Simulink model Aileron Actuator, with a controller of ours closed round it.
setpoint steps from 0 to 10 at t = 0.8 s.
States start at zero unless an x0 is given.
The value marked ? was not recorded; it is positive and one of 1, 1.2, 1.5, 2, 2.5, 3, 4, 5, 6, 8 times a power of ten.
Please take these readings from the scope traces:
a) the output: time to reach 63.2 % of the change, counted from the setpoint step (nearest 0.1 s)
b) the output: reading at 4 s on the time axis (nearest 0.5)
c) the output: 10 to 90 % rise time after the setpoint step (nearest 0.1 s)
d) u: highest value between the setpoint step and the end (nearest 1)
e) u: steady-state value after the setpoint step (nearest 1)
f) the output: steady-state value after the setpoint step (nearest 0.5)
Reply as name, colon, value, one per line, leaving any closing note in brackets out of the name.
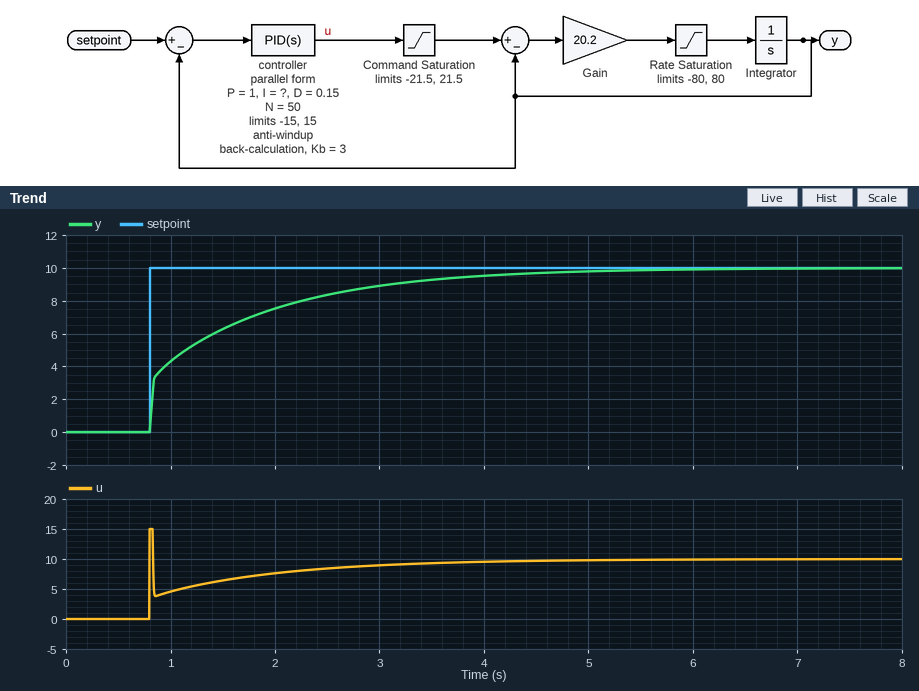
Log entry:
the output: time to reach 63.2 % of the change, counted from the setpoint step: 0.7 s
the output: reading at 4 s on the time axis: 9.5
the output: 10 to 90 % rise time after the setpoint step: 2.3 s
u: highest value between the setpoint step and the end: 15
u: steady-state value after the setpoint step: 10
the output: steady-state value after the setpoint step: 10.0
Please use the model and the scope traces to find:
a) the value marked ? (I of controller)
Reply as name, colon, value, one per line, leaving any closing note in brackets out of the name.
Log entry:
the value marked ?: 1.5
